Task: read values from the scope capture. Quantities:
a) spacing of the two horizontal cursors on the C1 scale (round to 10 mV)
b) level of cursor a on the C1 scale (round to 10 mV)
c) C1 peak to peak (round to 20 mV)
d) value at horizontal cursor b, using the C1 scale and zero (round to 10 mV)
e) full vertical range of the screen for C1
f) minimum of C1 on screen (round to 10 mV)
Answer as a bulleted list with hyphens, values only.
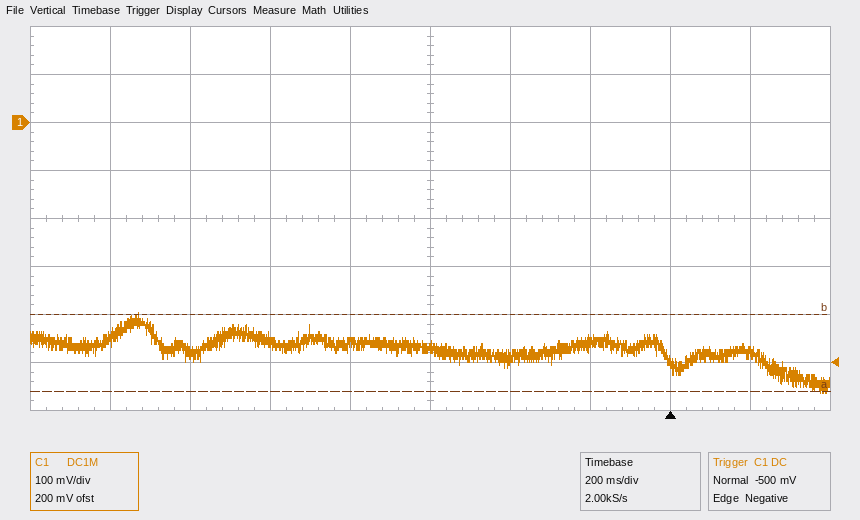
- 160 mV
- -560 mV
- 160 mV
- -400 mV
- 800 mV
- -560 mV
